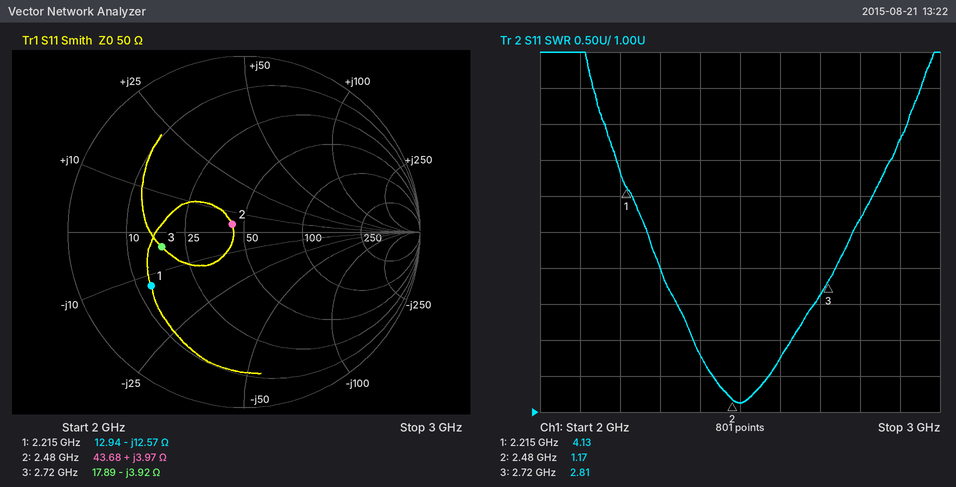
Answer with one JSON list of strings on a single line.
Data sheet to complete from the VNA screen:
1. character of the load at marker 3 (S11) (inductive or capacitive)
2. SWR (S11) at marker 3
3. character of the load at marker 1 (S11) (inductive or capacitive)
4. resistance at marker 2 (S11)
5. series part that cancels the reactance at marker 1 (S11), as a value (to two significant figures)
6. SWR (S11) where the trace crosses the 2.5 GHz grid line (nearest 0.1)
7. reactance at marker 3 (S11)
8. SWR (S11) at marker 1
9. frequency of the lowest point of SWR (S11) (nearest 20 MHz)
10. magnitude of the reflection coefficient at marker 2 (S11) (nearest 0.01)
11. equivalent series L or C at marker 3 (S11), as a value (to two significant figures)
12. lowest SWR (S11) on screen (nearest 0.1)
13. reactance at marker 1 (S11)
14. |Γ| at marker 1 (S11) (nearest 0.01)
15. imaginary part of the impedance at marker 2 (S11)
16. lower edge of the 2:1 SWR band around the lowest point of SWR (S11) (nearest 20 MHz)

["capacitive", "2.81", "capacitive", "43.68 Ω", "900 pH", "1.1", "-3.92 Ω", "4.13", "2.50 GHz", "0.08", "15 pF", "1.1", "-12.57 Ω", "0.61", "+3.97 Ω", "2.38 GHz"]
